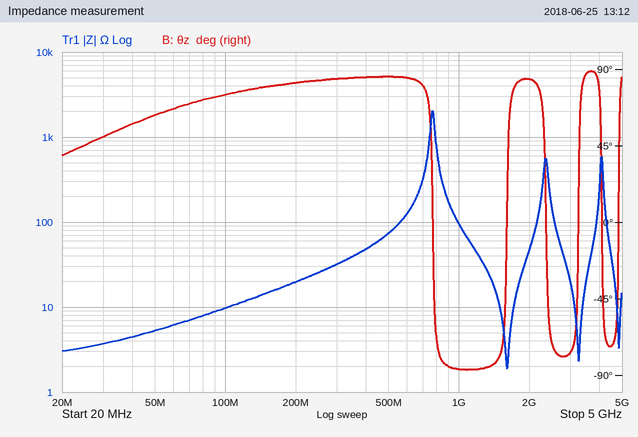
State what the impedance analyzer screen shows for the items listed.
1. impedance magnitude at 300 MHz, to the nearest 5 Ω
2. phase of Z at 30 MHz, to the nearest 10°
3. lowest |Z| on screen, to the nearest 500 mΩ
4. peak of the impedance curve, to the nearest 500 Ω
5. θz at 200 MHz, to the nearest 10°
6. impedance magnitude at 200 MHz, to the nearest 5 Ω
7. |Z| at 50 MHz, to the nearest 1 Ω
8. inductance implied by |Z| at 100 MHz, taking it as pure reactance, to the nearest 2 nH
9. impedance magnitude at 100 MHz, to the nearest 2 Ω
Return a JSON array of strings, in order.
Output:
["30 Ω", "50°", "2.0 Ω", "2.0 kΩ", "80°", "20 Ω", "5 Ω", "16 nH", "10 Ω"]
